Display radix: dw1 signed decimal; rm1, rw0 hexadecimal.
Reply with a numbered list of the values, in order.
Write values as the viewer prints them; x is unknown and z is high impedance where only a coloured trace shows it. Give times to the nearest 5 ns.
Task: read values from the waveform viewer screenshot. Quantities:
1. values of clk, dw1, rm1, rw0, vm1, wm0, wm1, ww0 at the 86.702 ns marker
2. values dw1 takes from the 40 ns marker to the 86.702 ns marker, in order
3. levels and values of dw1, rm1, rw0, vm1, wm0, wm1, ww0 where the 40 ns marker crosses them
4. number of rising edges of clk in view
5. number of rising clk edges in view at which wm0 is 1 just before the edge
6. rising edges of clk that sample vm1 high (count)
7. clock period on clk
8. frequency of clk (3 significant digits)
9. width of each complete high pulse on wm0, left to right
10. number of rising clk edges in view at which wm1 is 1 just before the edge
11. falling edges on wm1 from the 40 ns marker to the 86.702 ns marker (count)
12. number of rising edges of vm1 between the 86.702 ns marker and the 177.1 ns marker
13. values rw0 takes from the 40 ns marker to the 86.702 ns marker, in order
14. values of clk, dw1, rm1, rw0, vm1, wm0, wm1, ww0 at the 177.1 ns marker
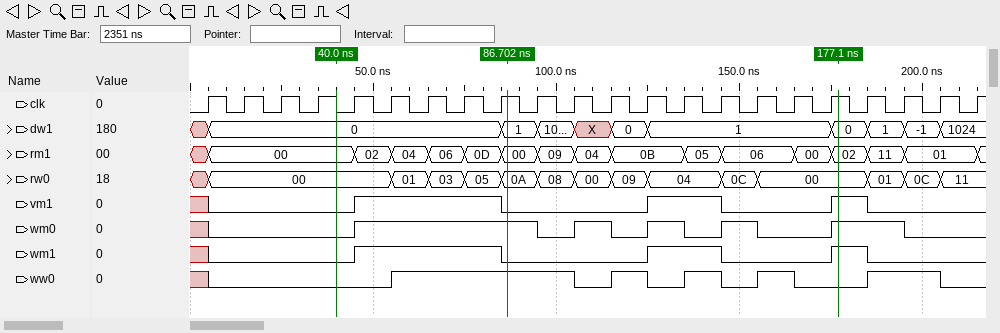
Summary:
1. clk=1, dw1=1, rm1=00, rw0=0A, vm1=0, wm0=1, wm1=0, ww0=1
2. 0, 1
3. dw1=0, rm1=00, rw0=00, vm1=0, wm0=0, wm1=0, ww0=0
4. 22
5. 10
6. 7
7. 10 ns
8. 100 MHz
9. 50 ns, 10 ns, 10 ns, 10 ns, 20 ns
10. 7
11. 1
12. 2
13. 00, 01, 03, 05, 0A
14. clk=1, dw1=0, rm1=02, rw0=00, vm1=1, wm0=1, wm1=1, ww0=0
